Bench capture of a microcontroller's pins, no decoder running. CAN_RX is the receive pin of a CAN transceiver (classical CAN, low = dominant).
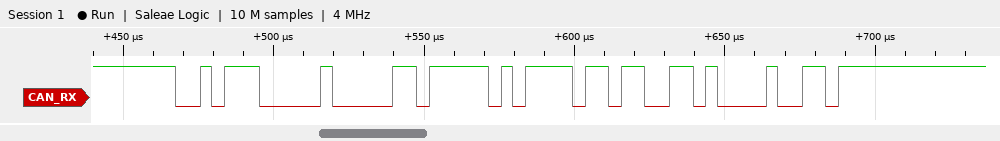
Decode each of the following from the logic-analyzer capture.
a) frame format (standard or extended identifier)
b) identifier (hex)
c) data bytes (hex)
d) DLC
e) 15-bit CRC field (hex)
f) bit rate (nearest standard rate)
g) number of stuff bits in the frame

standard
0x2E0
FD ED
2
0x4D09
250 kbit/s
3
